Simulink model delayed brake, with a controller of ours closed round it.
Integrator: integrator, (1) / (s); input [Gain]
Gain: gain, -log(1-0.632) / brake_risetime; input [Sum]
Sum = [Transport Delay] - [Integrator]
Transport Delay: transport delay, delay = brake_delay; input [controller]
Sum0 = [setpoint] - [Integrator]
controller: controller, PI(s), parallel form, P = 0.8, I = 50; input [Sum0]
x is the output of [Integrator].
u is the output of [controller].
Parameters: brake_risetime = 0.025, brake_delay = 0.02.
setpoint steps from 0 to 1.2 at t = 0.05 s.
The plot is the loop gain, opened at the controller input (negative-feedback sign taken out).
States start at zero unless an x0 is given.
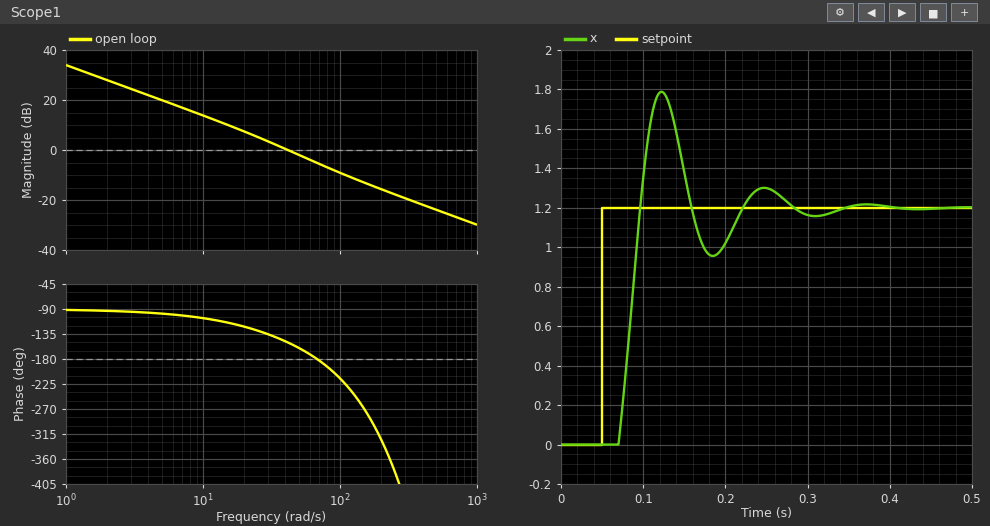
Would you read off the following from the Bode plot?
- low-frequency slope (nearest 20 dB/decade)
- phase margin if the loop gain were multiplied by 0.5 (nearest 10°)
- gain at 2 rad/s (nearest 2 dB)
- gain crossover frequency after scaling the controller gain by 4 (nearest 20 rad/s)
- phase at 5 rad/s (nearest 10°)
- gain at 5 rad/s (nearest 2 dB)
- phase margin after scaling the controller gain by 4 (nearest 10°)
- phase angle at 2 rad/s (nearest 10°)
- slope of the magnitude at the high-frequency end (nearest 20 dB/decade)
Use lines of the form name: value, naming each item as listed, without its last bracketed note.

low-frequency slope: -20 dB/decade
phase margin if the loop gain were multiplied by 0.5: 50°
gain at 2 rad/s: 28 dB
gain crossover frequency after scaling the controller gain by 4: 140 rad/s
phase at 5 rad/s: -100°
gain at 5 rad/s: 20 dB
phase margin after scaling the controller gain by 4: -70°
phase angle at 2 rad/s: -90°
slope of the magnitude at the high-frequency end: -20 dB/decade
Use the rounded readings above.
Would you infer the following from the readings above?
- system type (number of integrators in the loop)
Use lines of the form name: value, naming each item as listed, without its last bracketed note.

system type: 1
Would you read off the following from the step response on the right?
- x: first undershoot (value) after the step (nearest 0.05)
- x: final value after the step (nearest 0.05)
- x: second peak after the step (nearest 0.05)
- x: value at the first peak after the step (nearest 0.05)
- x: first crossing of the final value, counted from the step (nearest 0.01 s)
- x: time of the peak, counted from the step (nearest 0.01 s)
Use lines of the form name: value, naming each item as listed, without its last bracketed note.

x: first undershoot (value) after the step: 0.95
x: final value after the step: 1.20
x: second peak after the step: 1.30
x: value at the first peak after the step: 1.80
x: first crossing of the final value, counted from the step: 0.05 s
x: time of the peak, counted from the step: 0.07 s
